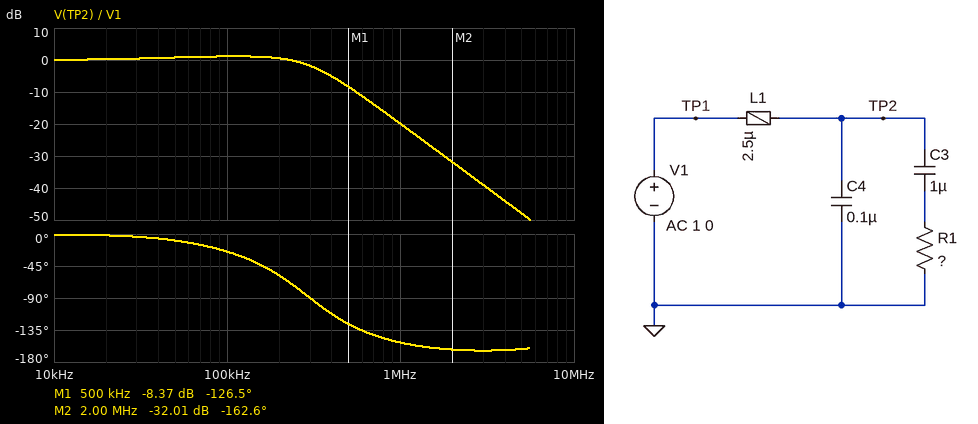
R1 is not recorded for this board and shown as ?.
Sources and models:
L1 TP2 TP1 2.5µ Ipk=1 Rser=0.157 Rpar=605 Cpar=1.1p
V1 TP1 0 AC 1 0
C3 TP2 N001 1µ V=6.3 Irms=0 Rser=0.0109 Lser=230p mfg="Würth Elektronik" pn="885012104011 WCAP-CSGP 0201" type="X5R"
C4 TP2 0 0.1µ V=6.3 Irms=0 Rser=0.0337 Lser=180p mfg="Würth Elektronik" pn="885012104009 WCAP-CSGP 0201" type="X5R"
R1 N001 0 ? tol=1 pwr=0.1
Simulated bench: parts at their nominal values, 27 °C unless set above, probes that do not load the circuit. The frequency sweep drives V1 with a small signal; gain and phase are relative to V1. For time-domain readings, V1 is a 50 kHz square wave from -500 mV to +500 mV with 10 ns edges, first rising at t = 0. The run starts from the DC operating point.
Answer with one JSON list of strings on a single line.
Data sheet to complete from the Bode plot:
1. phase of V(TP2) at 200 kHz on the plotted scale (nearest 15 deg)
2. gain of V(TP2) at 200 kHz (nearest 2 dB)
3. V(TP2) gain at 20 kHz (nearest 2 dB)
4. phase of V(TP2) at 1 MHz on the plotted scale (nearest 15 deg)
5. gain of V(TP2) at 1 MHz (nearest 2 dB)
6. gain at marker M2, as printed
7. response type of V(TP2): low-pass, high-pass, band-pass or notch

["-60 deg", "0 dB", "0 dB", "-150 deg", "-20 dB", "-32.01 dB", "low-pass"]
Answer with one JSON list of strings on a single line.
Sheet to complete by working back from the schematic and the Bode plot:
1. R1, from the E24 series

["3.9 Ω"]
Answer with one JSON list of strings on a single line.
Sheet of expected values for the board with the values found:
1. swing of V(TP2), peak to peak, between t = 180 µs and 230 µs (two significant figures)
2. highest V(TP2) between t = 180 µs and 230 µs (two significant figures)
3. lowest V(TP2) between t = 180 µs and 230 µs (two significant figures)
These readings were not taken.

["1.3 V", "660 mV", "-660 mV"]
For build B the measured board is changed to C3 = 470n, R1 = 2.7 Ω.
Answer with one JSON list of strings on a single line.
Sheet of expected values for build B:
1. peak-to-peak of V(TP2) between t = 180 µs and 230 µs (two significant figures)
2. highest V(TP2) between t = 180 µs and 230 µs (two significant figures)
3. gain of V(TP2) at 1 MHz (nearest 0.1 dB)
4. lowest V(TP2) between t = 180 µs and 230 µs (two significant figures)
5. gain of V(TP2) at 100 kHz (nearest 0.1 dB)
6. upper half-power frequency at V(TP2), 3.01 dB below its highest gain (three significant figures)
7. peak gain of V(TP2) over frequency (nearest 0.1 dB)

["1.7 V", "830 mV", "-21.0 dB", "-830 mV", "3.2 dB", "205 kHz", "3.7 dB"]
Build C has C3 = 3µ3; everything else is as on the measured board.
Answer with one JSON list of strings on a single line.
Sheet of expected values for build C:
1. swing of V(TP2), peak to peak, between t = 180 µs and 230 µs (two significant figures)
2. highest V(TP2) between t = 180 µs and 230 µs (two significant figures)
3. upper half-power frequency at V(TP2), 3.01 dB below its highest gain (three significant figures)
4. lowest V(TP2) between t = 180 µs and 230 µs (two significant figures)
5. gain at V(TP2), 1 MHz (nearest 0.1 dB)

["1.1 V", "570 mV", "333 kHz", "-570 mV", "-19.9 dB"]
